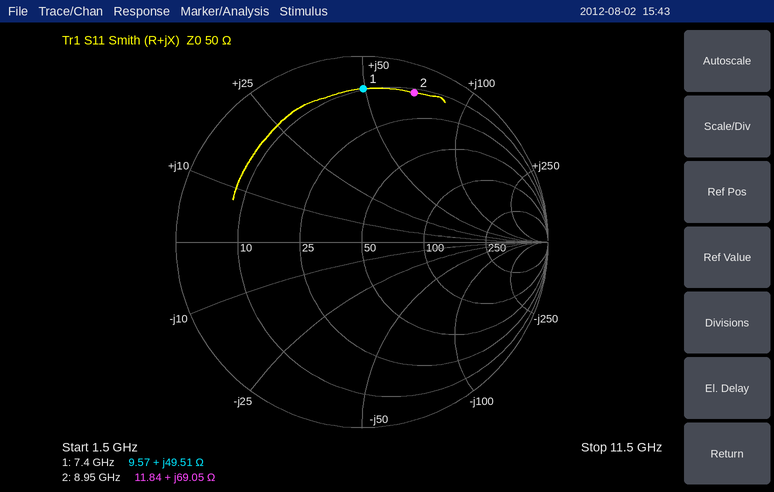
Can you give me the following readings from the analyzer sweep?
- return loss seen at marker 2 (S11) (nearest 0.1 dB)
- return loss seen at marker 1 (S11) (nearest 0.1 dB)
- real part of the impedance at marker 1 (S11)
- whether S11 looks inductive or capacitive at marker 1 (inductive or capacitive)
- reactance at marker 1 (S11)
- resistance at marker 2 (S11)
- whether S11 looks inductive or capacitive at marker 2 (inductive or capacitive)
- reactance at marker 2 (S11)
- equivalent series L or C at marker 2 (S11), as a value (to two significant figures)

1.4 dB
1.7 dB
9.57 Ω
inductive
+49.51 Ω
11.84 Ω
inductive
+69.05 Ω
1.2 nH
